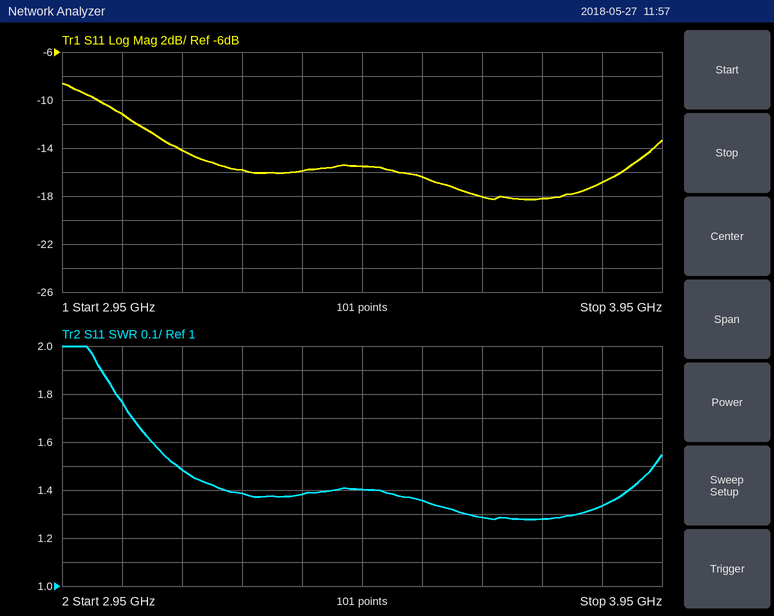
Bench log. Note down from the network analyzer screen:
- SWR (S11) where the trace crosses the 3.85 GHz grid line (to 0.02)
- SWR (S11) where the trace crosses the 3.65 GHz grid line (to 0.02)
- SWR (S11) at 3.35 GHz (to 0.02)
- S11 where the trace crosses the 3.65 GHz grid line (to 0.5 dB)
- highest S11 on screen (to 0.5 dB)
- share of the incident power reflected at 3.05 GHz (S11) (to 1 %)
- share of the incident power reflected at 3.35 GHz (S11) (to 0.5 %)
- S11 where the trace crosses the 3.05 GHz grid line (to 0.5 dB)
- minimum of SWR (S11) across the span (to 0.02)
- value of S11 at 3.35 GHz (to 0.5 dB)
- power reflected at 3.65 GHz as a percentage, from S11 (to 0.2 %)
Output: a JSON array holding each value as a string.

["1.34", "1.28", "1.38", "-18.0 dB", "-8.5 dB", "8 %", "2.5 %", "-11.0 dB", "1.28", "-16.0 dB", "1.6 %"]
